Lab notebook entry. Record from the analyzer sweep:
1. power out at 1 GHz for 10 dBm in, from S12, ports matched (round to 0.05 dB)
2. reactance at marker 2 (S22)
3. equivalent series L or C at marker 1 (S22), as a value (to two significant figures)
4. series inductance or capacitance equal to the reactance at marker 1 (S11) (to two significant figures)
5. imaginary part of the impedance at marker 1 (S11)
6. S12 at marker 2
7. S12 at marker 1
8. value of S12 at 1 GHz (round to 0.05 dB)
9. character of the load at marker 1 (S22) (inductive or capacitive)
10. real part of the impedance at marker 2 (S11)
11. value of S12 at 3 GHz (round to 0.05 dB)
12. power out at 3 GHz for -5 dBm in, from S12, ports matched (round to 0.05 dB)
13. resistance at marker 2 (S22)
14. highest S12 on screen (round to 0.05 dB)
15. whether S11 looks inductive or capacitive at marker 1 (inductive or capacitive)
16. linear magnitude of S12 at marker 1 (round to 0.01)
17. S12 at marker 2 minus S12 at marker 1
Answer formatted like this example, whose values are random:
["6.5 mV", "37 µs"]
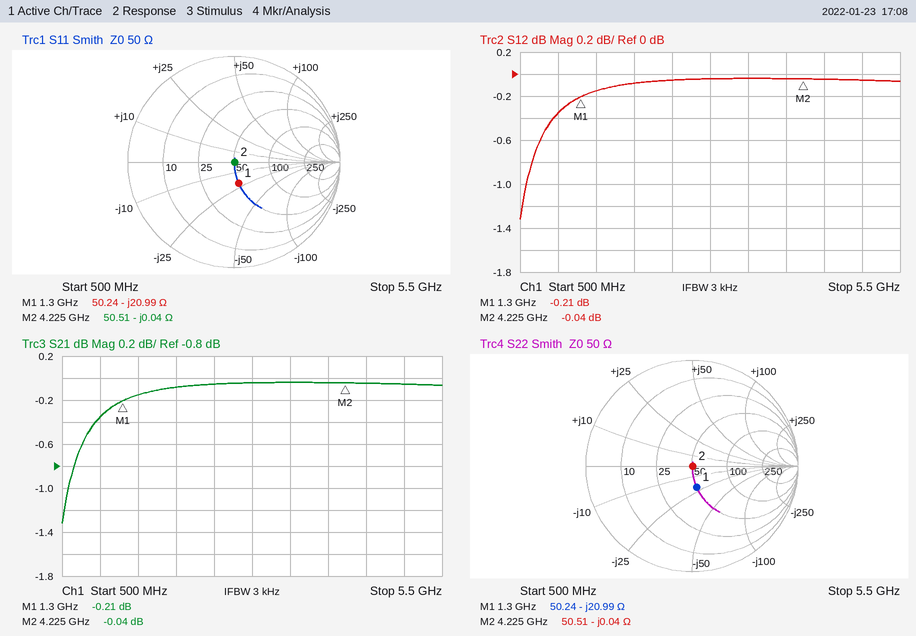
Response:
["9.65 dBm", "-0.04 Ω", "5.8 pF", "5.8 pF", "-20.99 Ω", "-0.04 dB", "-0.21 dB", "-0.35 dB", "capacitive", "50.51 Ω", "-0.05 dB", "-5.05 dBm", "50.51 Ω", "-0.05 dB", "capacitive", "0.98", "0.17 dB"]
